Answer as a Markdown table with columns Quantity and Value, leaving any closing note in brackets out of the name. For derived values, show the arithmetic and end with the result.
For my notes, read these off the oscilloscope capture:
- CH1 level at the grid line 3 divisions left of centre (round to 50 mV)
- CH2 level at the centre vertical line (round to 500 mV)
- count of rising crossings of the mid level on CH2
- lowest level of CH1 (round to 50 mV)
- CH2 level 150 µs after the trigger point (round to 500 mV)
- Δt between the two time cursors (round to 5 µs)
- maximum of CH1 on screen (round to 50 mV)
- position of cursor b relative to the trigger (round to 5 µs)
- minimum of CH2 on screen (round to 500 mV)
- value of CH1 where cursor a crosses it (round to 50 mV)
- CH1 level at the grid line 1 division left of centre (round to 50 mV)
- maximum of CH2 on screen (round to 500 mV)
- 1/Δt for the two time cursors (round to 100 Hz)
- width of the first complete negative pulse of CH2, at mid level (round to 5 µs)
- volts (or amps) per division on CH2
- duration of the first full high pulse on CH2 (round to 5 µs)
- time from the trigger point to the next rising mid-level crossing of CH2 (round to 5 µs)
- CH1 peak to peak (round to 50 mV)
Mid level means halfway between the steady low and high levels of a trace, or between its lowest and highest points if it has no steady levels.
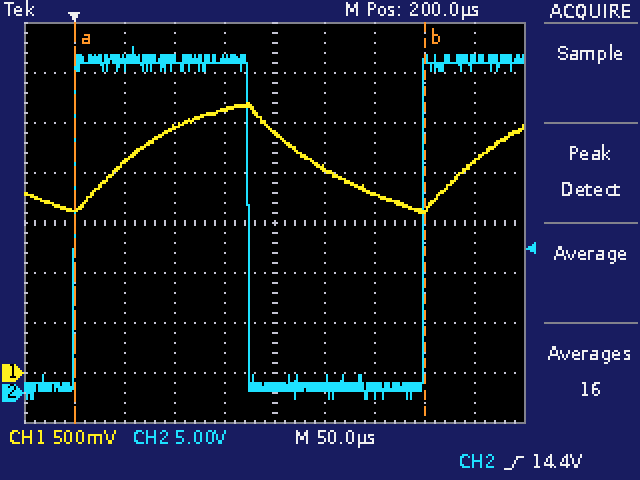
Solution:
| Quantity | Value |
|---|---|
| CH1 level at the grid line 3 divisions left of centre | 2.10 V |
| CH2 level at the centre vertical line | 500 mV |
| count of rising crossings of the mid level on CH2 | 2 |
| lowest level of CH1 | 1.60 V |
| CH2 level 150 µs after the trigger point | 33.5 V |
| Δt between the two time cursors | 350 µs |
| maximum of CH1 on screen | 2.70 V |
| position of cursor b relative to the trigger | +350 µs |
| minimum of CH2 on screen | -500 mV |
| value of CH1 where cursor a crosses it | 1.65 V |
| CH1 level at the grid line 1 division left of centre | 2.65 V |
| maximum of CH2 on screen | 34.5 V |
| 1/Δt for the two time cursors | 1 / 350 µs ≈ 2.9 kHz |
| width of the first complete negative pulse of CH2, at mid level | 175 µs |
| volts (or amps) per division on CH2 | 5 V |
| duration of the first full high pulse on CH2 | 175 µs |
| time from the trigger point to the next rising mid-level crossing of CH2 | 350 µs |
| CH1 peak to peak | 2.70 V − (1.60 V) = 1.10 V |
